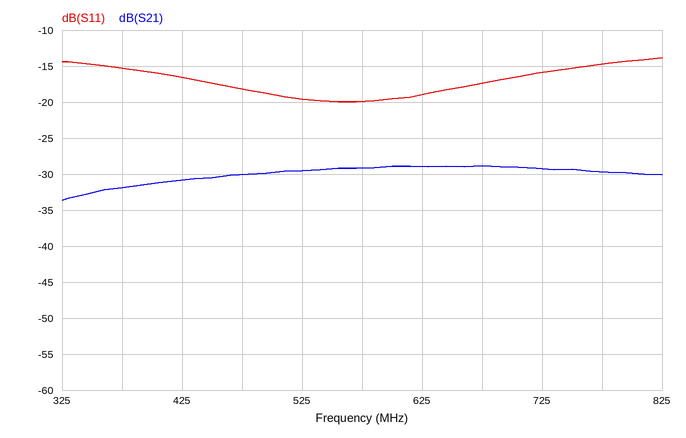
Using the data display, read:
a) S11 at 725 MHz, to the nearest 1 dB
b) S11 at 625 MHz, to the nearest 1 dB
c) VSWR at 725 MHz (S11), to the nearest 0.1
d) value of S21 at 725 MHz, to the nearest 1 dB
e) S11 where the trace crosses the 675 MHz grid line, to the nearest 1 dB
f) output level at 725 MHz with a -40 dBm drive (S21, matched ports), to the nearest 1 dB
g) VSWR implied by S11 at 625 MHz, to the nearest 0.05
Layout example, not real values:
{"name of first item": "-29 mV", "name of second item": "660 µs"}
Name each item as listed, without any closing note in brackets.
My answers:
{"S11 at 725 MHz, to the nearest 1 dB": "-16 dB", "S11 at 625 MHz, to the nearest 1 dB": "-19 dB", "VSWR at 725 MHz (S11), to the nearest 0.1": "1.4", "value of S21 at 725 MHz, to the nearest 1 dB": "-29 dB", "S11 where the trace crosses the 675 MHz grid line, to the nearest 1 dB": "-17 dB", "output level at 725 MHz with a -40 dBm drive (S21, matched ports), to the nearest 1 dB": "-69 dBm", "VSWR implied by S11 at 625 MHz, to the nearest 0.05": "1.25"}
